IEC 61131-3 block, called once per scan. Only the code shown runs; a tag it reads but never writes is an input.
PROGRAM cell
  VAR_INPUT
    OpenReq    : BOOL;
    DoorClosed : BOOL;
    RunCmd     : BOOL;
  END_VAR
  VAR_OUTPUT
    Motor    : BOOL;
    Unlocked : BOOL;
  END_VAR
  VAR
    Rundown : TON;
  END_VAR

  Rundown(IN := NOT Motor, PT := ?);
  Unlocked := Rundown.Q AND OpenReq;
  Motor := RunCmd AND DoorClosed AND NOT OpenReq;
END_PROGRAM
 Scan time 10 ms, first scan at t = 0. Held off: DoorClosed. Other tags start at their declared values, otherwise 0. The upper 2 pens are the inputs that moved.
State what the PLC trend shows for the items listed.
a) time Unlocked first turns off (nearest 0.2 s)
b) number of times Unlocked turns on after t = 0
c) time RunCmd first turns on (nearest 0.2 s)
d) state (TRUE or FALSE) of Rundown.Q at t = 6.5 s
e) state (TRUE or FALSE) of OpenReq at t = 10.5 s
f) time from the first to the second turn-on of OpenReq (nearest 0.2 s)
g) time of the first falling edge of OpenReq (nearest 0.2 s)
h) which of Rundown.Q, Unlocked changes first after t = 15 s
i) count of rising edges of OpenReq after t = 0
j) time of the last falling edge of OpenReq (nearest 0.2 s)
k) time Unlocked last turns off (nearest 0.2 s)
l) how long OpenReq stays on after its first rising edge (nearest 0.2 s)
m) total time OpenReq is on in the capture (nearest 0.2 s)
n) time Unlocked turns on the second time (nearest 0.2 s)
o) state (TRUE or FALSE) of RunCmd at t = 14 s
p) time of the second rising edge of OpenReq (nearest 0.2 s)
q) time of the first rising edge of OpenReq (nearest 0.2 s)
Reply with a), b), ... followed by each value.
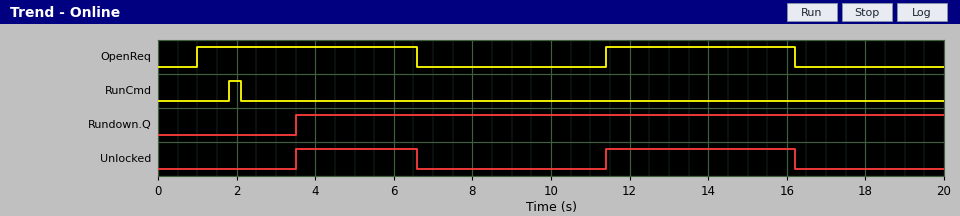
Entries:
a) 6.6 s
b) 2
c) 1.8 s
d) TRUE
e) FALSE
f) 10.4 s
g) 6.6 s
h) Unlocked
i) 2
j) 16.2 s
k) 16.2 s
l) 5.6 s
m) 10.4 s
n) 11.4 s
o) FALSE
p) 11.4 s
q) 1.0 s
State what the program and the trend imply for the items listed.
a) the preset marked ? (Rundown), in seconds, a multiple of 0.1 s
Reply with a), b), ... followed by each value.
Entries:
a) 3.5 s
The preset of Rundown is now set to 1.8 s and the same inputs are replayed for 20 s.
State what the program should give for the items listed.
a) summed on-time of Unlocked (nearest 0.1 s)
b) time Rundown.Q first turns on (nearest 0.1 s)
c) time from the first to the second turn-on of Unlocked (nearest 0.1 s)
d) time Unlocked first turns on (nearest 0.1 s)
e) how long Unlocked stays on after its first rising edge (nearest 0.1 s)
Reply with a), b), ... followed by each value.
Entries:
a) 9.6 s
b) 1.8 s
c) 9.6 s
d) 1.8 s
e) 4.8 s
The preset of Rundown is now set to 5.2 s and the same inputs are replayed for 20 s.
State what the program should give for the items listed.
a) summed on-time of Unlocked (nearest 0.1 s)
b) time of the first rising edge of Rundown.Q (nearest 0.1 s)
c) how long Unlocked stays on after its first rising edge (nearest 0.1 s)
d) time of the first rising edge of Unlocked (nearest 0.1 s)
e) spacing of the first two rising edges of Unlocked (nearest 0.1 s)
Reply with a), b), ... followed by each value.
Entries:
a) 6.2 s
b) 5.2 s
c) 1.4 s
d) 5.2 s
e) 6.2 s
